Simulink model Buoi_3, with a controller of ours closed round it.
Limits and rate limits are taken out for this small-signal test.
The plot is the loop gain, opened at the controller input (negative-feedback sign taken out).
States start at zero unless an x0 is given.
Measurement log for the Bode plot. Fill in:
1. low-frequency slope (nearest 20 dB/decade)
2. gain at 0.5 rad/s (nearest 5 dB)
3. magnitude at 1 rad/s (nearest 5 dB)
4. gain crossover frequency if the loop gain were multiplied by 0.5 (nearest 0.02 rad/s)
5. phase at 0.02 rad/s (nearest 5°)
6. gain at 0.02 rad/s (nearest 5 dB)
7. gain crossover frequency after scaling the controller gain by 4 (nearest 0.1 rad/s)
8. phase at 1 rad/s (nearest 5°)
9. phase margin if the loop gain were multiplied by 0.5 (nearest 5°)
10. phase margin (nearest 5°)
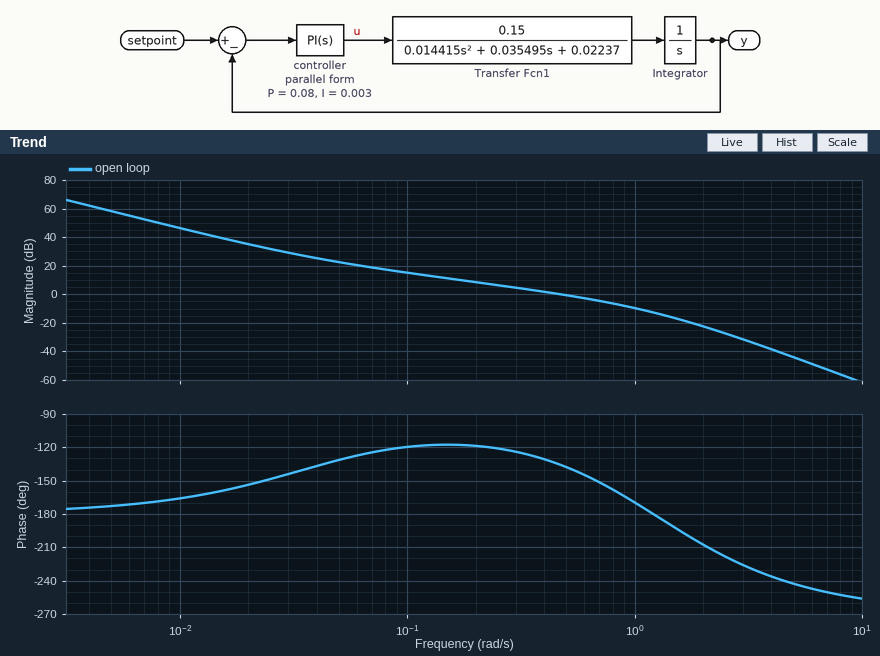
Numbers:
-40 dB/decade
0 dB
-10 dB
0.26 rad/s
-155°
35 dB
1.2 rad/s
-170°
60°
45°
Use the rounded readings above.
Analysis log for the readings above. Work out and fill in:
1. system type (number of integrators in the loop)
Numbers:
2
